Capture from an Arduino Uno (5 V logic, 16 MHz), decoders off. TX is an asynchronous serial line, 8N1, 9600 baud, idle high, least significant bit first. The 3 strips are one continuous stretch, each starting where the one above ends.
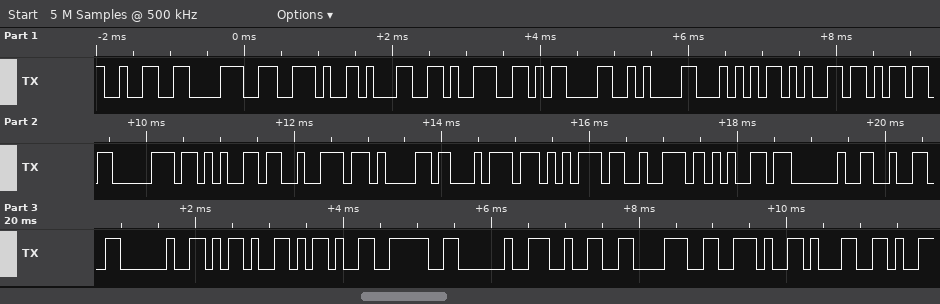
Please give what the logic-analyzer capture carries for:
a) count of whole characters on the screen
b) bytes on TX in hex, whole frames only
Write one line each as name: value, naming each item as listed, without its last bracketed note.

count of whole characters on the screen: 29
bytes on TX in hex, whole frames only: 32 38 2E 31 39 0D 0A 54 65 6D 70 65 72 61 74 75 72 65 20 32 20 2D 2D 3E 20 32 38 2E 31
